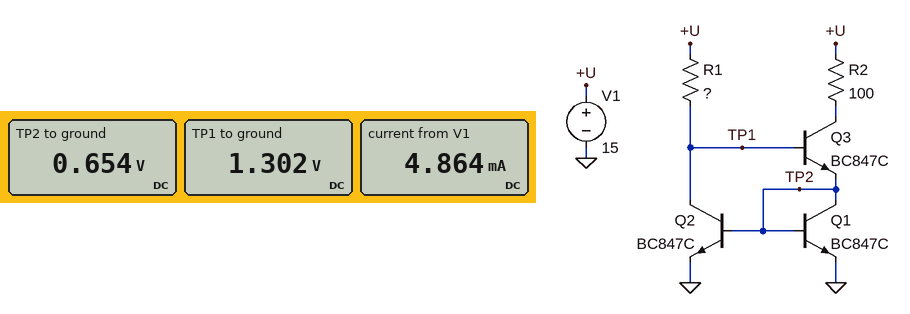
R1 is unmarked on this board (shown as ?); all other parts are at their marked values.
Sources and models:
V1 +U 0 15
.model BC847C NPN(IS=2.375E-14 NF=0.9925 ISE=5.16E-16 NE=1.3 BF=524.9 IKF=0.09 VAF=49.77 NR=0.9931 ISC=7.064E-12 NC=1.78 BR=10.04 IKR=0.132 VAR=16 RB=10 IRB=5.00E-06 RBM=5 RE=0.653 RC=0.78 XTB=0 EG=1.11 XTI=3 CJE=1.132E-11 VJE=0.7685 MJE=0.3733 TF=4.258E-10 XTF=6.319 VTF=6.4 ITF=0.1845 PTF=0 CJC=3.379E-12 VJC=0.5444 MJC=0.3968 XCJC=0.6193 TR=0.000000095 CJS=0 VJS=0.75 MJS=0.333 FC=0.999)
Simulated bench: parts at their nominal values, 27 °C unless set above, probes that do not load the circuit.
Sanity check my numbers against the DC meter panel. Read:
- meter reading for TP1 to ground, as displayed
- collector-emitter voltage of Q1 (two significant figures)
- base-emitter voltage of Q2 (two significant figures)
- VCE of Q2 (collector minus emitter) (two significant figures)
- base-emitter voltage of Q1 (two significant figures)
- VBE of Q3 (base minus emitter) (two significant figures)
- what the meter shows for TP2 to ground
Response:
1.302 V
650 mV
650 mV
1.3 V
650 mV
650 mV
0.654 V
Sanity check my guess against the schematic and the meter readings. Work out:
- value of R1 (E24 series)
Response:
5.6 kΩ
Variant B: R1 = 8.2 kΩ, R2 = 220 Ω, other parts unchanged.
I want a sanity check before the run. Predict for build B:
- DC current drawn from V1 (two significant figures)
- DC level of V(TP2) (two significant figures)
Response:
3.3 mA
640 mV
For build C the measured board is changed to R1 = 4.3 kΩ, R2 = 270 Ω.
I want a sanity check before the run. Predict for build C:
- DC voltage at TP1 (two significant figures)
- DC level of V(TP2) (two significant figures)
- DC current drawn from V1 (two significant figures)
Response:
1.3 V
660 mV
6.3 mA
